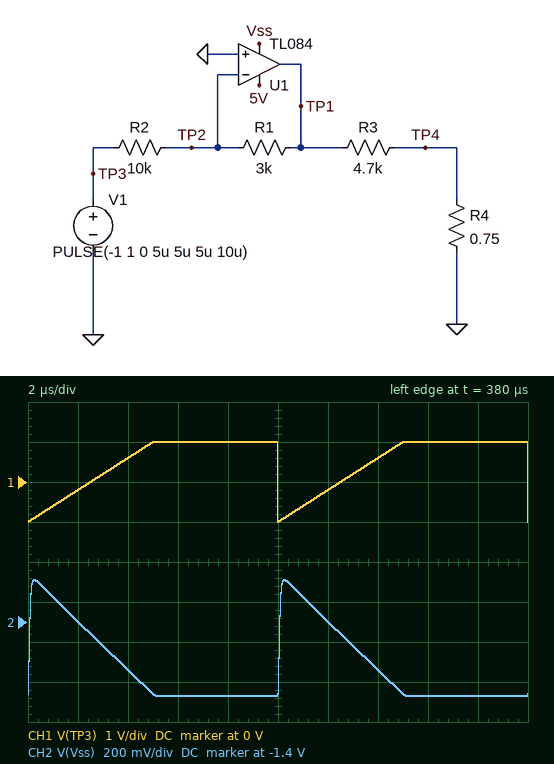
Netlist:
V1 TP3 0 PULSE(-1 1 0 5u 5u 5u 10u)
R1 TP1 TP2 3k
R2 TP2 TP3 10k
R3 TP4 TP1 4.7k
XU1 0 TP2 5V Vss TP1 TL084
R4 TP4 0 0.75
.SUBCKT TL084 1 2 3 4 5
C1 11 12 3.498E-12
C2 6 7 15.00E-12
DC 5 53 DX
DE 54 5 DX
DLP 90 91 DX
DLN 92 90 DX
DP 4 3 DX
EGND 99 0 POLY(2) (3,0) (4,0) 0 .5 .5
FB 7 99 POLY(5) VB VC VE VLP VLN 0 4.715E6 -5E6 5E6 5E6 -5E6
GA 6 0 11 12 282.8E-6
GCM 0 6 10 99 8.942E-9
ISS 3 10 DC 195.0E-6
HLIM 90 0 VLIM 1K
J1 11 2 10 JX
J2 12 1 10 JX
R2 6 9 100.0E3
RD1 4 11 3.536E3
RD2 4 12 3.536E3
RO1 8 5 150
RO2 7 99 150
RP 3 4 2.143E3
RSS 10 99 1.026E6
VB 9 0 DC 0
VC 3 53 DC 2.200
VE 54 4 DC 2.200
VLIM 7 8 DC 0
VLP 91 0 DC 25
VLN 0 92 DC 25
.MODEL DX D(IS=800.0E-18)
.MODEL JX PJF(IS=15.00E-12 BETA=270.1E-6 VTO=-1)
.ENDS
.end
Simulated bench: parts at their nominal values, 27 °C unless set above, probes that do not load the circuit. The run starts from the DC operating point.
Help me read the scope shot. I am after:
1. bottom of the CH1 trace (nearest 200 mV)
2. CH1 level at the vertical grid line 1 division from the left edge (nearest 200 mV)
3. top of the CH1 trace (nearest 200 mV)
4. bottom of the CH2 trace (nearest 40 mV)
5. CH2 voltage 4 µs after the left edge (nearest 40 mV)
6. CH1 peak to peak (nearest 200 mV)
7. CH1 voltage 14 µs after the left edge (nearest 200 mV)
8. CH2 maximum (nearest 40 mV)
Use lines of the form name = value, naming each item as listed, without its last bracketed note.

bottom of the CH1 trace = -1.0 V
CH1 level at the vertical grid line 1 division from the left edge = -200 mV
top of the CH1 trace = 1.0 V
bottom of the CH2 trace = -1.76 V
CH2 voltage 4 µs after the left edge = -1.64 V
CH1 peak to peak = 2.0 V
CH1 voltage 14 µs after the left edge = 600 mV
CH2 maximum = -1.20 V
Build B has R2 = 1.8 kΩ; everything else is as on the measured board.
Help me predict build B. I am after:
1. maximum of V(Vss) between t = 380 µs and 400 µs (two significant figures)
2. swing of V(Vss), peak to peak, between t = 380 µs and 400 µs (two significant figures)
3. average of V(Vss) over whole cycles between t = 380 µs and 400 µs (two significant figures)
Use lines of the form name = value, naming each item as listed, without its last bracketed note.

maximum of V(Vss) between t = 380 µs and 400 µs = -500 mV
swing of V(Vss), peak to peak, between t = 380 µs and 400 µs = 2.6 V
average of V(Vss) over whole cycles between t = 380 µs and 400 µs = -2.3 V
